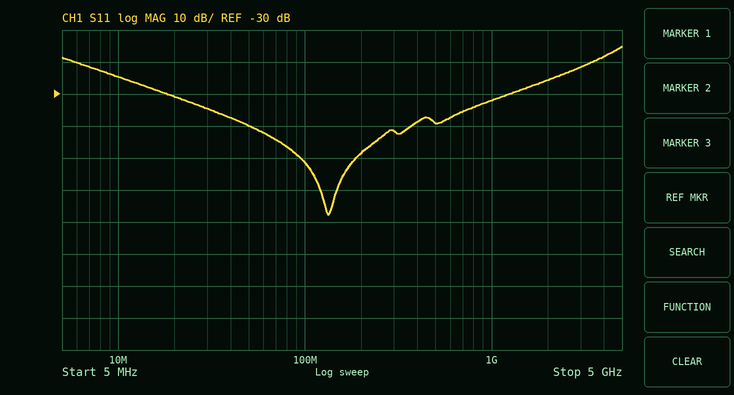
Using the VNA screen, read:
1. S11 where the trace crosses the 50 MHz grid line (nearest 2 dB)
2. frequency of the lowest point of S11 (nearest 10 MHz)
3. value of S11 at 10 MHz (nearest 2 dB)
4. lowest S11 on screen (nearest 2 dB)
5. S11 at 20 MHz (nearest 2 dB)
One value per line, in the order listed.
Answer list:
-40 dB
130 MHz
-24 dB
-68 dB
-30 dB
